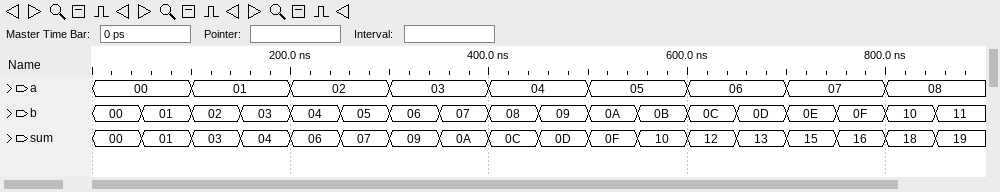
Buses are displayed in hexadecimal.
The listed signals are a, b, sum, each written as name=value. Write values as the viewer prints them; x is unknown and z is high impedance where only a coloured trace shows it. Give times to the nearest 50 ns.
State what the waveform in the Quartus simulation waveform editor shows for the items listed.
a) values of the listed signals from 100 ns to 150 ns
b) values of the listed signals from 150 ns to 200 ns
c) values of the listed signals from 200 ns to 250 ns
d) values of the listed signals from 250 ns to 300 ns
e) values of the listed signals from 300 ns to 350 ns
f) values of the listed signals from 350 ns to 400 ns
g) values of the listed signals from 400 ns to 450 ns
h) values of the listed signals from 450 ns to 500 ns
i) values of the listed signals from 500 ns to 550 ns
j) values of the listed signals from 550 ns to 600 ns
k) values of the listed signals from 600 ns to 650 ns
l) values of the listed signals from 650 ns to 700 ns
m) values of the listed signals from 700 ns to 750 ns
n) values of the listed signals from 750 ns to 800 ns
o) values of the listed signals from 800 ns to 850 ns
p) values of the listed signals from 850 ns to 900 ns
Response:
a=01, b=02, sum=03
a=01, b=03, sum=04
a=02, b=04, sum=06
a=02, b=05, sum=07
a=03, b=06, sum=09
a=03, b=07, sum=0A
a=04, b=08, sum=0C
a=04, b=09, sum=0D
a=05, b=0A, sum=0F
a=05, b=0B, sum=10
a=06, b=0C, sum=12
a=06, b=0D, sum=13
a=07, b=0E, sum=15
a=07, b=0F, sum=16
a=08, b=10, sum=18
a=08, b=11, sum=19
